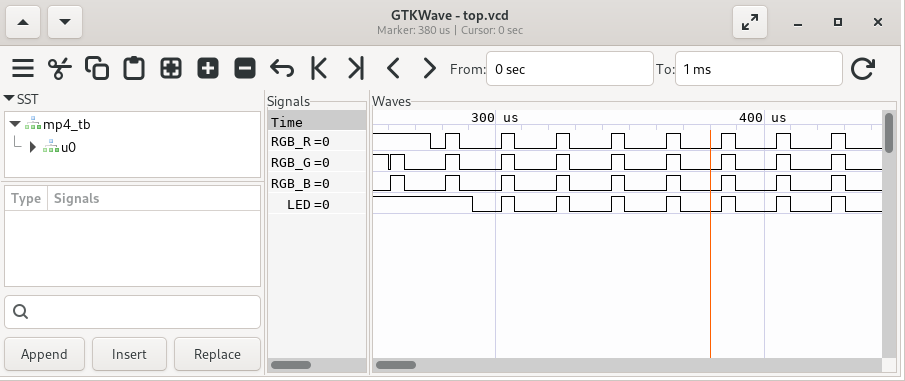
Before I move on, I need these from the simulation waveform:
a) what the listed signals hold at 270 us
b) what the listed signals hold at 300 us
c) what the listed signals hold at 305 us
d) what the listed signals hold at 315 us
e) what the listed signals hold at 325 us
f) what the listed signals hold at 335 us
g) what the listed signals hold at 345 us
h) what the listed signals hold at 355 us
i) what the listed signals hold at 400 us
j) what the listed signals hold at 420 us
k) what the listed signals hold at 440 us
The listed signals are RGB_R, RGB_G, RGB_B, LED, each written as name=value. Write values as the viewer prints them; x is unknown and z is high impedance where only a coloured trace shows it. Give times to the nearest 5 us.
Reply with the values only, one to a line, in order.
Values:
RGB_R=1, RGB_G=0, RGB_B=0, LED=1
RGB_R=0, RGB_G=0, RGB_B=0, LED=0
RGB_R=1, RGB_G=1, RGB_B=1, LED=1
RGB_R=0, RGB_G=0, RGB_B=0, LED=0
RGB_R=1, RGB_G=1, RGB_B=1, LED=1
RGB_R=0, RGB_G=0, RGB_B=0, LED=0
RGB_R=1, RGB_G=1, RGB_B=1, LED=1
RGB_R=0, RGB_G=0, RGB_B=0, LED=0
RGB_R=0, RGB_G=0, RGB_B=0, LED=0
RGB_R=0, RGB_G=0, RGB_B=0, LED=0
RGB_R=0, RGB_G=0, RGB_B=0, LED=0
